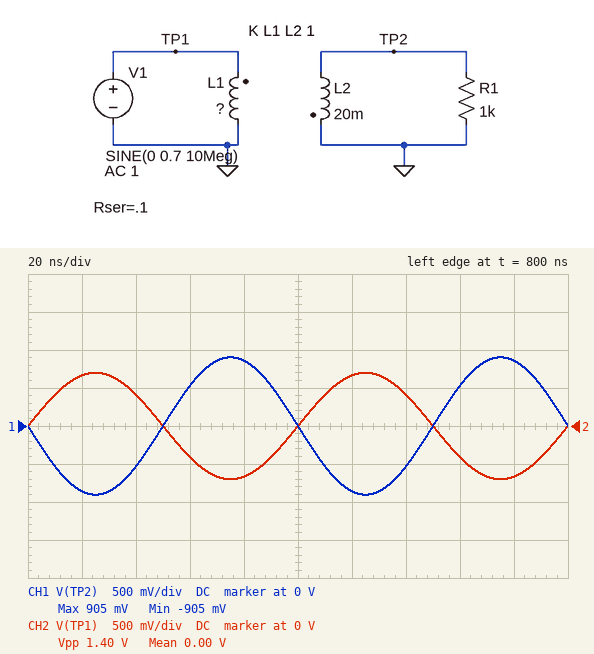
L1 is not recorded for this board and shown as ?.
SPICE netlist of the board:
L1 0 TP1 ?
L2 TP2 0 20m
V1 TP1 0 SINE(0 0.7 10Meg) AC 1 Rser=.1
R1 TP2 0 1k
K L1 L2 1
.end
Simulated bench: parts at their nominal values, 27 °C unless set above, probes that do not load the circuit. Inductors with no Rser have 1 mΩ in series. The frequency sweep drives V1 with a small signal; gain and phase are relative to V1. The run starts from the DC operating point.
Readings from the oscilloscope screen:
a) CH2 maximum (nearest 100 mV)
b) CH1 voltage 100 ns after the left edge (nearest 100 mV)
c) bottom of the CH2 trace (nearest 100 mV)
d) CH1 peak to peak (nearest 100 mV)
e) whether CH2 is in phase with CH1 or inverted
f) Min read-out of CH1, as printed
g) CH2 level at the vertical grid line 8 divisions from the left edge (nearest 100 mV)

700 mV
0 V
-700 mV
1.8 V
inverted
-905 mV
-400 mV
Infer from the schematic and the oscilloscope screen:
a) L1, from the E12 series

12 mH
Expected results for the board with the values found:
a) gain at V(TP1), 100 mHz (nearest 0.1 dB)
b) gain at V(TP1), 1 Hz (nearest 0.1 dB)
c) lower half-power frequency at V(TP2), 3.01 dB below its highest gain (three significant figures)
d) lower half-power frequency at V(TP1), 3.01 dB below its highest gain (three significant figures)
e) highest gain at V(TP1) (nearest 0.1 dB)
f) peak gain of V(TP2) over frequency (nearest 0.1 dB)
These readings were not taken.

-22.5 dB
-4.5 dB
1.34 Hz
1.34 Hz
0 dB
2.2 dB
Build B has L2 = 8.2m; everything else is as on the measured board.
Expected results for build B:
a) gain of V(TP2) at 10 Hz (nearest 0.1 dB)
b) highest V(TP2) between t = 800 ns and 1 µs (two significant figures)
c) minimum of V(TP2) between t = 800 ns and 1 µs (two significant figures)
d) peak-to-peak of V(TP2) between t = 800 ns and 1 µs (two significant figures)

-1.7 dB
580 mV
-580 mV
1.2 V
